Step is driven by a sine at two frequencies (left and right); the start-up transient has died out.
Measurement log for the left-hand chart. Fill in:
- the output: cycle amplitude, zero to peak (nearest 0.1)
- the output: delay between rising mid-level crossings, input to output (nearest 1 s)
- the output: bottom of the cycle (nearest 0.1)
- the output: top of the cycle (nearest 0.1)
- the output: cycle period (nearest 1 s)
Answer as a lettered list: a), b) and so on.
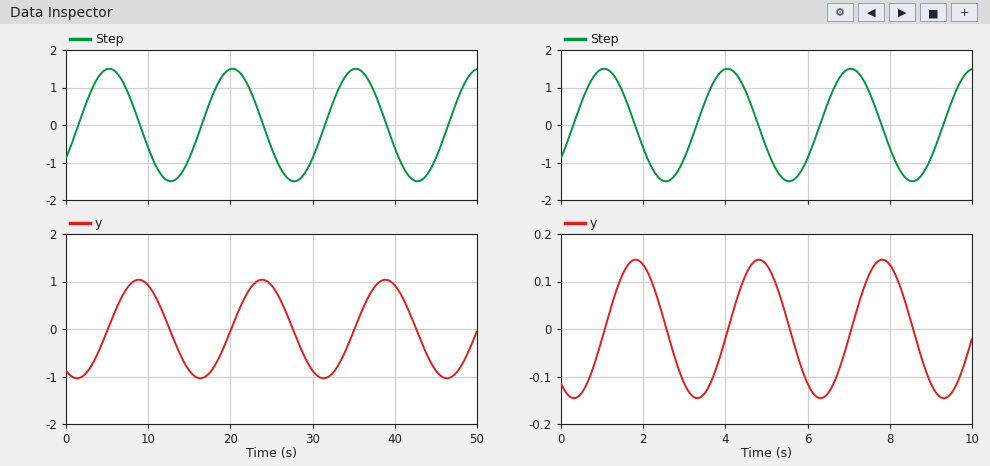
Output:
a) 1.0
b) 4 s
c) -1.0
d) 1.0
e) 15 s
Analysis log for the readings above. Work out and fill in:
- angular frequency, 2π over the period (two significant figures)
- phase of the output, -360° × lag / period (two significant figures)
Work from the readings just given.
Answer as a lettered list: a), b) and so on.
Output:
a) 0.42 rad/s
b) -96°
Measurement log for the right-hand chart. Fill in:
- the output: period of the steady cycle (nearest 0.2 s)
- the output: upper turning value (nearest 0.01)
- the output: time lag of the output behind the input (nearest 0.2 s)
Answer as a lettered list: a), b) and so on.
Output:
a) 3.0 s
b) 0.15
c) 0.8 s
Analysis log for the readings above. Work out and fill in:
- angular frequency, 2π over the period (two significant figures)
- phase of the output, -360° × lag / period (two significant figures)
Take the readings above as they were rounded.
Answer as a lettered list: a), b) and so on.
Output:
a) 2.1 rad/s
b) -96°
